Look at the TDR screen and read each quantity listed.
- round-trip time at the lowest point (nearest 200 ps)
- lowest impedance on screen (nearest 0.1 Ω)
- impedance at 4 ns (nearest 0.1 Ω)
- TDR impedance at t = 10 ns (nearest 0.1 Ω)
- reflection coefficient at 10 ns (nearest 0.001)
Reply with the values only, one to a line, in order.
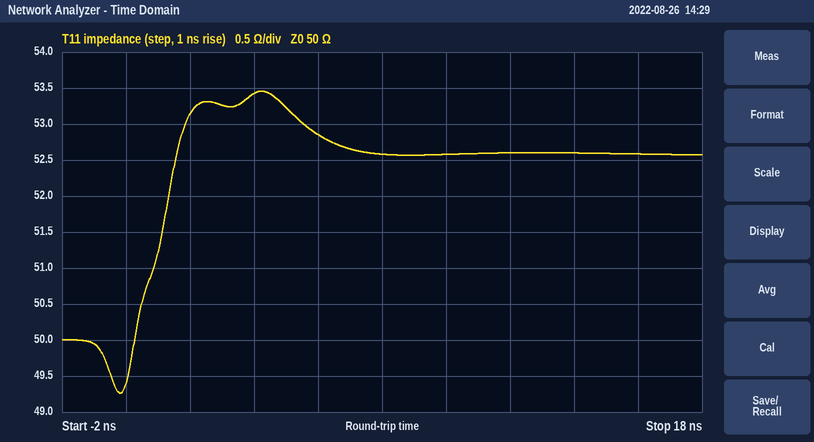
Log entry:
-200 ps
49.3 Ω
53.4 Ω
52.6 Ω
+0.025
